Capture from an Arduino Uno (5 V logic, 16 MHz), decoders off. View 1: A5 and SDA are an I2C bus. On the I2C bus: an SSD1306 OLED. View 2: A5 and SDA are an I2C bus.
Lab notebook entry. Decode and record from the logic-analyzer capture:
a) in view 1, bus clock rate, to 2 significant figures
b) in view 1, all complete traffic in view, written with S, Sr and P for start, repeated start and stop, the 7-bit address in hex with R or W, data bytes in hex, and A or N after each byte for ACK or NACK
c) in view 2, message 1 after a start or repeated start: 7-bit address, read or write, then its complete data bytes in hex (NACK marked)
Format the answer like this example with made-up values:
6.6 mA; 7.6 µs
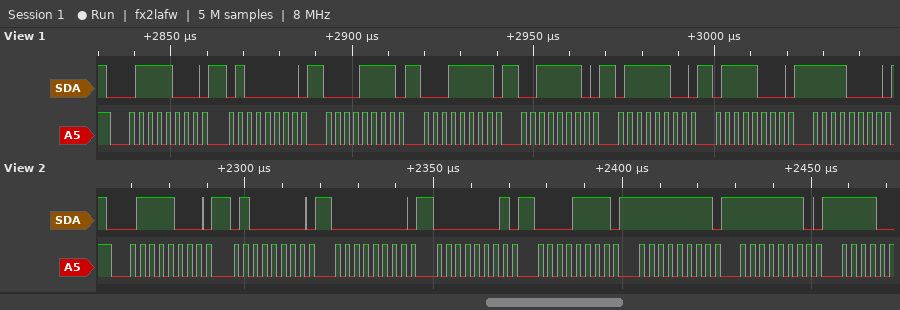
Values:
400 kHz; S 3CW A 40 A 0F A 1F A 3E A 7C A 78 A F0 A; 0x3C write: 40 00 01 0F FF FE
